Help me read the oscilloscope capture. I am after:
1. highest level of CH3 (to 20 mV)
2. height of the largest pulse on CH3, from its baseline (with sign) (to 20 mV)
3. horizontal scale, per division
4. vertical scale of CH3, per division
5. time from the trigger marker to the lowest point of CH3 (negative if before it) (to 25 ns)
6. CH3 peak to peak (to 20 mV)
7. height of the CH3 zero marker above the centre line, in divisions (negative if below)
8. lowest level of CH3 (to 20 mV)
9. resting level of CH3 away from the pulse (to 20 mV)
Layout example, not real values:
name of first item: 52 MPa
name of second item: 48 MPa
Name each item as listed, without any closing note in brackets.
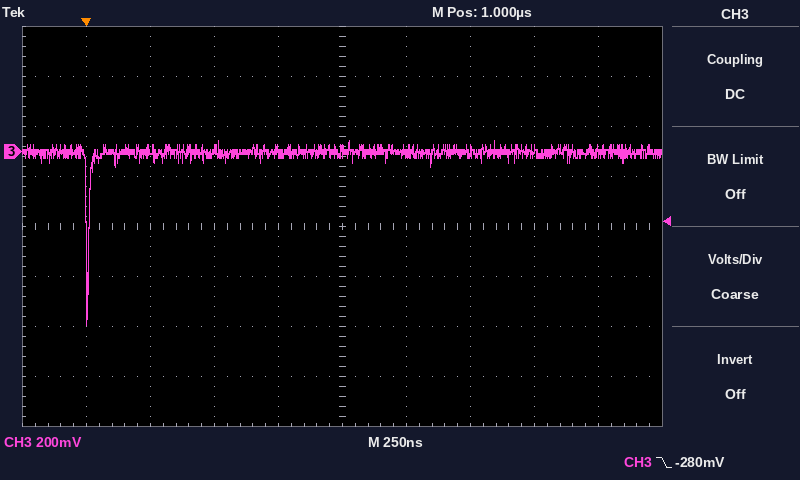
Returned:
highest level of CH3: 40 mV
height of the largest pulse on CH3, from its baseline (with sign): -700 mV
horizontal scale, per division: 250 ns
vertical scale of CH3, per division: 200 mV
time from the trigger marker to the lowest point of CH3 (negative if before it): 0 ns
CH3 peak to peak: 740 mV
height of the CH3 zero marker above the centre line, in divisions: +1.5 div
lowest level of CH3: -700 mV
resting level of CH3 away from the pulse: 0 mV
